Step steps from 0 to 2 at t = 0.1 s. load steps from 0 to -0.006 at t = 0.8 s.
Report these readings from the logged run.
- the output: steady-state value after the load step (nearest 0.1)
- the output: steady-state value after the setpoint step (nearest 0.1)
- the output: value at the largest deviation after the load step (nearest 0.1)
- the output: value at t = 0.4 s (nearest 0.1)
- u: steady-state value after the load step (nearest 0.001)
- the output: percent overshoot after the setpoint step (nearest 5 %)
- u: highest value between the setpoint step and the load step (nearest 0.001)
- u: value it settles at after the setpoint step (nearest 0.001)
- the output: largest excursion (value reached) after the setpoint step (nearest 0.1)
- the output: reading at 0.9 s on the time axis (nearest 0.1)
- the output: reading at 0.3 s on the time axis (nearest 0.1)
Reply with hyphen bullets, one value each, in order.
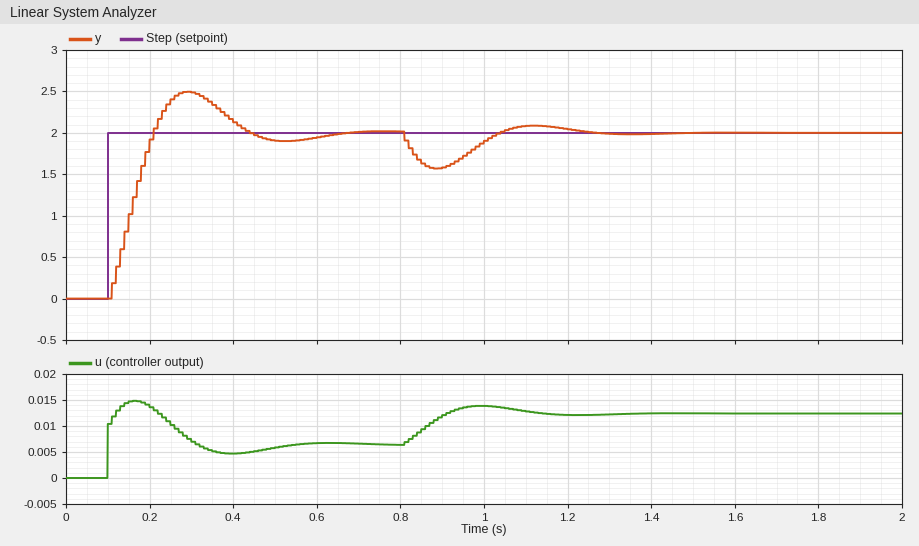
- 2.0
- 2.0
- 1.6
- 2.1
- 0.012
- 25 %
- 0.015
- 0.006
- 2.5
- 1.6
- 2.5
